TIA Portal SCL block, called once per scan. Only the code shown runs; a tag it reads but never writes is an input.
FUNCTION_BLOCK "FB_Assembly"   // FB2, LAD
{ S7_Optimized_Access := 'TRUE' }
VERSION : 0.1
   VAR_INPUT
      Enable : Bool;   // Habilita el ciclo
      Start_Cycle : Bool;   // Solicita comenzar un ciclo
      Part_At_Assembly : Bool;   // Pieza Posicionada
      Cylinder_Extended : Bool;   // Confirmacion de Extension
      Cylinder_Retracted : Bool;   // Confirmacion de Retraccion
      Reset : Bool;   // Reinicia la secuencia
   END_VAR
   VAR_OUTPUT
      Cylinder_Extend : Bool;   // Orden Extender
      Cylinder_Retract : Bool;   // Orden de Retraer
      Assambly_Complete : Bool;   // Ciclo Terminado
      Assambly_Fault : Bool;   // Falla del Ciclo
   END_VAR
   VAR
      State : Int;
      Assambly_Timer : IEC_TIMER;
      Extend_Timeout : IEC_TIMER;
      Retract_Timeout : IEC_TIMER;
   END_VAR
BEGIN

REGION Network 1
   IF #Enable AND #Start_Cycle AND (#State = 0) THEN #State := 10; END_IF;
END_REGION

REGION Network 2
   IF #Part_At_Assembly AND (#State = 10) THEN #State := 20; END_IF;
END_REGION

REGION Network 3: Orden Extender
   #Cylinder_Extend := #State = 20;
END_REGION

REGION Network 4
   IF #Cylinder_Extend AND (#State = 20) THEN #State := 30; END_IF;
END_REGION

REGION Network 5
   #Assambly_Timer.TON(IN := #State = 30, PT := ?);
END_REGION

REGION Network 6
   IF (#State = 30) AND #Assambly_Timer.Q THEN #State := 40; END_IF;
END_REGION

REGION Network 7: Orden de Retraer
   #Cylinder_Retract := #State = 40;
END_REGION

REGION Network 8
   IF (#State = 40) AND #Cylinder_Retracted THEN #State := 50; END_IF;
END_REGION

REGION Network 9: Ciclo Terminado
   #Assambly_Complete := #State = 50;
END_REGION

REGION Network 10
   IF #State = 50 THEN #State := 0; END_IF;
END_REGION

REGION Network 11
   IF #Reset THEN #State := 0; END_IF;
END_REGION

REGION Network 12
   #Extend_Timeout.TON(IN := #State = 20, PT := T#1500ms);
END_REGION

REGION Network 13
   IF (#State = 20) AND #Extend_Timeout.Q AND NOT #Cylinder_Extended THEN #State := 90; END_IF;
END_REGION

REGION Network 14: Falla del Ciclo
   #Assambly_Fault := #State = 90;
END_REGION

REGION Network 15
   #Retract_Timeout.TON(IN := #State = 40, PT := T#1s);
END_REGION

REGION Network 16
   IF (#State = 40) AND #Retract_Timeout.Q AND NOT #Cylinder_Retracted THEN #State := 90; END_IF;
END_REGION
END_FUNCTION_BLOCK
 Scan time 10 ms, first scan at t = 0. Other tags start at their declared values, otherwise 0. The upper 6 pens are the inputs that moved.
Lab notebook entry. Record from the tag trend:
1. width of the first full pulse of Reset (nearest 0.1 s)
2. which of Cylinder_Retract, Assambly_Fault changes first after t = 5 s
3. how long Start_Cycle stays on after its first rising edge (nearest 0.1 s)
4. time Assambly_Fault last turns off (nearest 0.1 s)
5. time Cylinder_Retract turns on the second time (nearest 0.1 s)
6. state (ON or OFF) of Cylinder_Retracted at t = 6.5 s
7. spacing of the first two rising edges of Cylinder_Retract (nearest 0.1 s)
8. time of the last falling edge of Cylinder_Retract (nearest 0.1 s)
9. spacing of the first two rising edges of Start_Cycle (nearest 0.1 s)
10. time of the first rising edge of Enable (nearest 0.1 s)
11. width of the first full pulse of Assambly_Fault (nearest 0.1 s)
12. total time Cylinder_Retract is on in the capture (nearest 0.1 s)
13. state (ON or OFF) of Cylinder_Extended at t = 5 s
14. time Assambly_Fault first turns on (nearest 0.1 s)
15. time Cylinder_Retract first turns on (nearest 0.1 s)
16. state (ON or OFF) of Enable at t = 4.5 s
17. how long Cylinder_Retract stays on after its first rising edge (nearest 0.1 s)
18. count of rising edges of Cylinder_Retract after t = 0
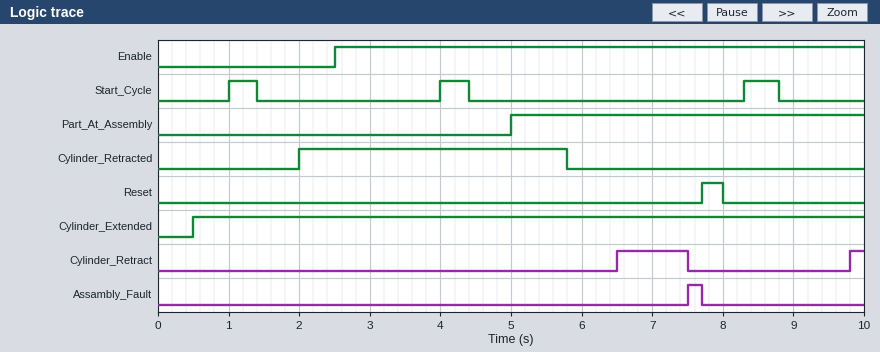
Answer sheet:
0.3 s
Cylinder_Retract
0.4 s
7.7 s
9.8 s
OFF
3.3 s
7.5 s
3.0 s
2.5 s
0.2 s
1.2 s
ON
7.5 s
6.5 s
ON
1.0 s
2
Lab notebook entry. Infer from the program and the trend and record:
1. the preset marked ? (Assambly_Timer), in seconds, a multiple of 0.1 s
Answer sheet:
1.5 s
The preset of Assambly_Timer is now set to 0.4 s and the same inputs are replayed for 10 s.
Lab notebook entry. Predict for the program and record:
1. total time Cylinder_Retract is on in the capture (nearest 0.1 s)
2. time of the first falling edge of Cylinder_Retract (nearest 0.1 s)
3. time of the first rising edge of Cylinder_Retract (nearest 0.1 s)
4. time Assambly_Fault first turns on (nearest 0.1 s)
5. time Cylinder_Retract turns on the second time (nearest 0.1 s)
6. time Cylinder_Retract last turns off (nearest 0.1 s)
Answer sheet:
1.0 s
5.4 s
5.4 s
9.7 s
8.7 s
9.7 s
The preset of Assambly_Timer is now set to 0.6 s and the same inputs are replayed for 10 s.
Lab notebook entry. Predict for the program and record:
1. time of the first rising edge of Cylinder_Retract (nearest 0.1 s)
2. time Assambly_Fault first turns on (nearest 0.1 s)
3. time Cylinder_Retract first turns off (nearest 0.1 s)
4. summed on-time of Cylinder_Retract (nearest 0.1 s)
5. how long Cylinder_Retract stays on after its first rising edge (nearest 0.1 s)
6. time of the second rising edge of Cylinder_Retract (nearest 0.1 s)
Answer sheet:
5.6 s
9.9 s
5.6 s
1.0 s
0.0 s
8.9 s
